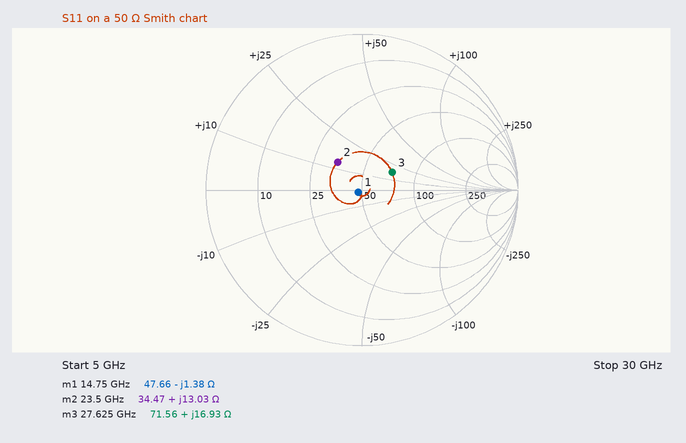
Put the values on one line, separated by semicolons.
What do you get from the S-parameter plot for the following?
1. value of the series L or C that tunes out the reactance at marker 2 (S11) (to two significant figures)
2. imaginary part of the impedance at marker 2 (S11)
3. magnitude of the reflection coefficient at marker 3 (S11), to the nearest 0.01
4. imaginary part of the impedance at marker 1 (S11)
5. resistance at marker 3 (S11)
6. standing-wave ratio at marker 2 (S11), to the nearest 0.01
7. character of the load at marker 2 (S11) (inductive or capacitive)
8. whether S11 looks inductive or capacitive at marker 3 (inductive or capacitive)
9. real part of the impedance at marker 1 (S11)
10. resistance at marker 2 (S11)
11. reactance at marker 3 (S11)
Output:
520 fF; +13.03 Ω; 0.22; -1.38 Ω; 71.56 Ω; 1.62; inductive; inductive; 47.66 Ω; 34.47 Ω; +16.93 Ω
